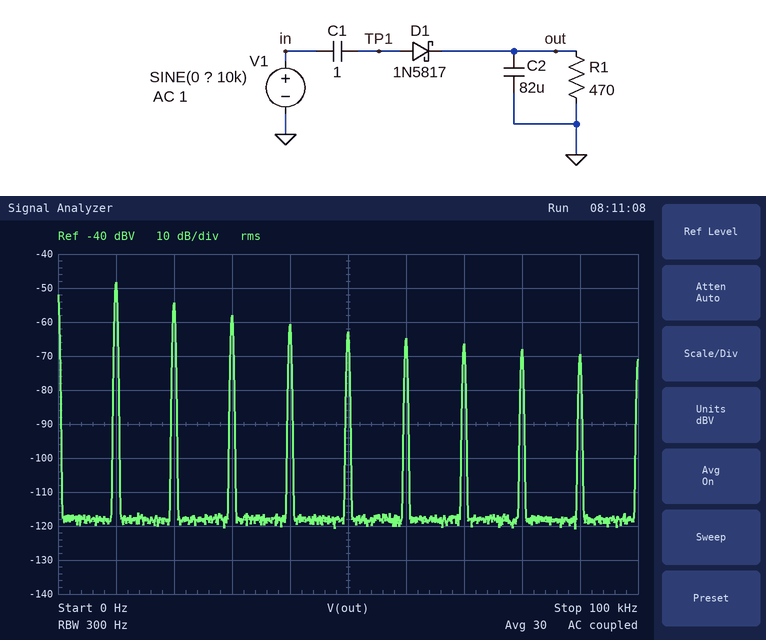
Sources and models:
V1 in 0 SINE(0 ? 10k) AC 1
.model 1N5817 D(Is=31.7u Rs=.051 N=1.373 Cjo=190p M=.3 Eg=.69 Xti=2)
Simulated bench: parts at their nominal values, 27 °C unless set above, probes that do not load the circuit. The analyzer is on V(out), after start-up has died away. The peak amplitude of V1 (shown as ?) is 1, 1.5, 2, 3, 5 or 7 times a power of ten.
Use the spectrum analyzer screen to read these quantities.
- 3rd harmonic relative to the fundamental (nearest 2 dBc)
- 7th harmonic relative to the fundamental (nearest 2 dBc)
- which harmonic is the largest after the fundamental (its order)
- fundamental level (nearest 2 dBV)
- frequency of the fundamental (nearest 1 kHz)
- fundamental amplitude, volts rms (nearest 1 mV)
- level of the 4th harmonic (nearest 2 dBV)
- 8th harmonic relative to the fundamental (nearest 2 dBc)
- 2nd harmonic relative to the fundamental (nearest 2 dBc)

-10 dBc
-18 dBc
2
-48 dBV
10 kHz
4 mV
-60 dBV
-20 dBc
-6 dBc
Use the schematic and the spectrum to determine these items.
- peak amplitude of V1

7 V
